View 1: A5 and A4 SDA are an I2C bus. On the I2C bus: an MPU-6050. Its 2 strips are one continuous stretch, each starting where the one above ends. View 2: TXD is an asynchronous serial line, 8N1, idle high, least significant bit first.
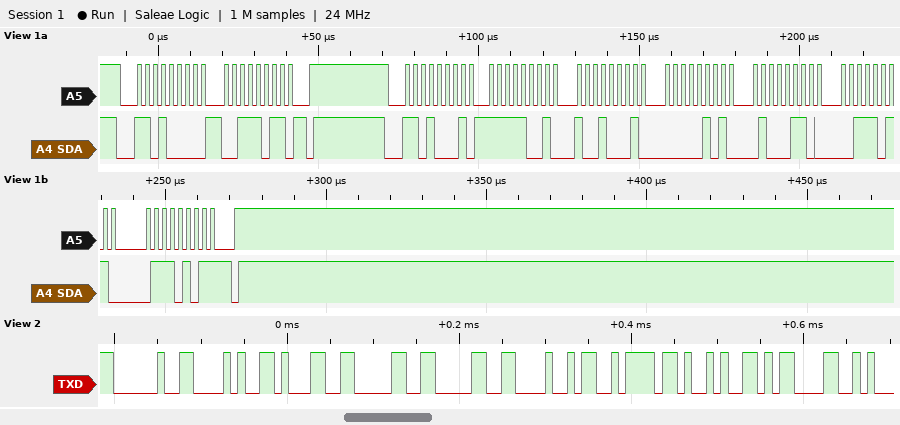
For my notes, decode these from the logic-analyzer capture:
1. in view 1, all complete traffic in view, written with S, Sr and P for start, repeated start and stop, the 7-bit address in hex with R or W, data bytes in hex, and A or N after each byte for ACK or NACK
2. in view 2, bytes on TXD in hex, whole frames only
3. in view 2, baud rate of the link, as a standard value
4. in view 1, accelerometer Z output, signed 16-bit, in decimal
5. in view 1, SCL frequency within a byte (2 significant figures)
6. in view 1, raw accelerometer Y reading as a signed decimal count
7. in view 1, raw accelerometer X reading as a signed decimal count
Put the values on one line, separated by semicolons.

S 68W A 3B A P S 68R A F9 A 91 A 05 A 46 A 3B A 75 N P; 0x20 0x28 0x31 0x30 0x30 0x48 0x7A 0x29 0x0D; 115200 baud; 15221; 400 kHz; 1350; -1647
